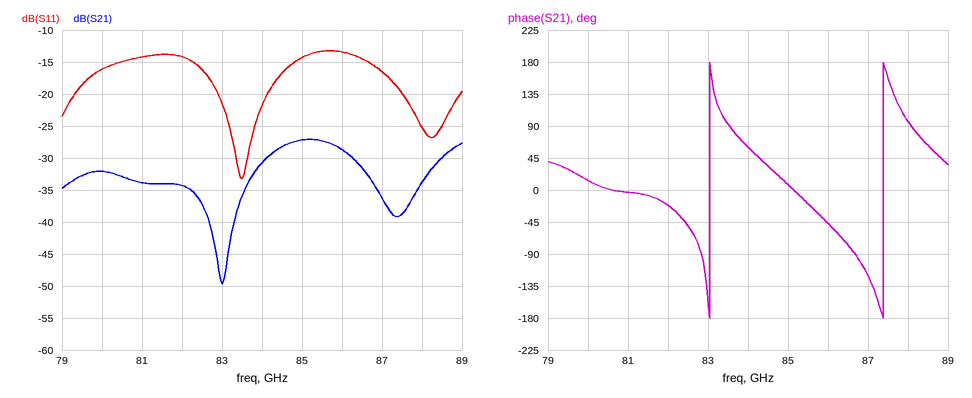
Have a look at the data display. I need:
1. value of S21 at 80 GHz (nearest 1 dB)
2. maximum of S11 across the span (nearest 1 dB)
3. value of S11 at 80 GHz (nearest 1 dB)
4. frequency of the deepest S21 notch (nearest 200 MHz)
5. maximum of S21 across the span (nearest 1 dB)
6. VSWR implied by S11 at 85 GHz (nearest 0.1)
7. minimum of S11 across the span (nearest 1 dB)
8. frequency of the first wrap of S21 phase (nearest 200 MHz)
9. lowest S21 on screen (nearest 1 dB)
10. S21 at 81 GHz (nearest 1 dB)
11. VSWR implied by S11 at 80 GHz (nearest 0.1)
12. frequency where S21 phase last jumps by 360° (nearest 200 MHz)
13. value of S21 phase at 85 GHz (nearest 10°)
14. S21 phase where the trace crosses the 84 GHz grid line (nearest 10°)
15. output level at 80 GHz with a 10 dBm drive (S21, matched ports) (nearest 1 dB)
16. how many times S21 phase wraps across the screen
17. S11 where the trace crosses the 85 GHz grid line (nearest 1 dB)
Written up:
-32 dB
-13 dB
-16 dB
83.0 GHz
-27 dB
1.5
-33 dB
83.0 GHz
-50 dB
-34 dB
1.4
87.4 GHz
10°
60°
-22 dBm
2
-14 dB
